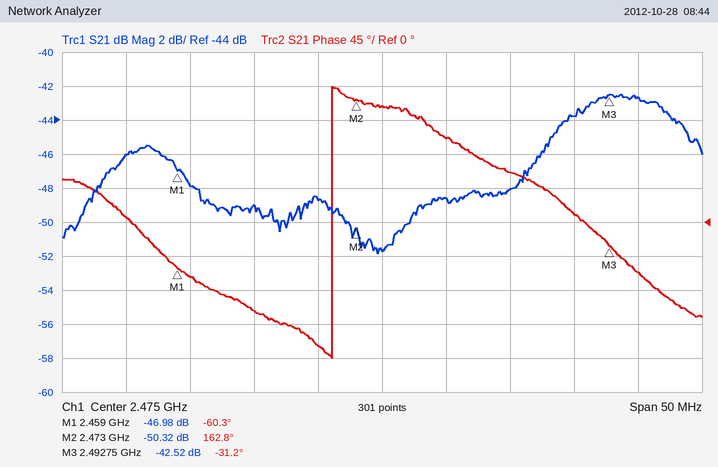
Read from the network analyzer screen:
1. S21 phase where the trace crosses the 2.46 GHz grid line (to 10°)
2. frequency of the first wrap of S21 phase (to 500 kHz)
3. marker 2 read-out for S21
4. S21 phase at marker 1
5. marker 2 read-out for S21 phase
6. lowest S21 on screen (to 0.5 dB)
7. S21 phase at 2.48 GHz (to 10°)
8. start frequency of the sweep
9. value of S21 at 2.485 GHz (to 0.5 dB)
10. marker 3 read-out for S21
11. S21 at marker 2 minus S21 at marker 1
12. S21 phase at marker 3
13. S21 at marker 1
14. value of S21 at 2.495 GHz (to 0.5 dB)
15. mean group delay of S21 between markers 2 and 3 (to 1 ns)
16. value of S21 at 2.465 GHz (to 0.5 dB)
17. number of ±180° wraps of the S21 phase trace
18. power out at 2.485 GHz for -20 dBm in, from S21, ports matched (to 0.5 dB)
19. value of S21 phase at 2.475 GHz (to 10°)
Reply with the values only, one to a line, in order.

-70°
2.4710 GHz
-50.32 dB
-60.3°
162.8°
-52.0 dB
110°
2.45 GHz
-48.0 dB
-42.52 dB
-3.34 dB
-31.2°
-46.98 dB
-42.5 dB
27 ns
-49.0 dB
1
-68.0 dBm
150°
